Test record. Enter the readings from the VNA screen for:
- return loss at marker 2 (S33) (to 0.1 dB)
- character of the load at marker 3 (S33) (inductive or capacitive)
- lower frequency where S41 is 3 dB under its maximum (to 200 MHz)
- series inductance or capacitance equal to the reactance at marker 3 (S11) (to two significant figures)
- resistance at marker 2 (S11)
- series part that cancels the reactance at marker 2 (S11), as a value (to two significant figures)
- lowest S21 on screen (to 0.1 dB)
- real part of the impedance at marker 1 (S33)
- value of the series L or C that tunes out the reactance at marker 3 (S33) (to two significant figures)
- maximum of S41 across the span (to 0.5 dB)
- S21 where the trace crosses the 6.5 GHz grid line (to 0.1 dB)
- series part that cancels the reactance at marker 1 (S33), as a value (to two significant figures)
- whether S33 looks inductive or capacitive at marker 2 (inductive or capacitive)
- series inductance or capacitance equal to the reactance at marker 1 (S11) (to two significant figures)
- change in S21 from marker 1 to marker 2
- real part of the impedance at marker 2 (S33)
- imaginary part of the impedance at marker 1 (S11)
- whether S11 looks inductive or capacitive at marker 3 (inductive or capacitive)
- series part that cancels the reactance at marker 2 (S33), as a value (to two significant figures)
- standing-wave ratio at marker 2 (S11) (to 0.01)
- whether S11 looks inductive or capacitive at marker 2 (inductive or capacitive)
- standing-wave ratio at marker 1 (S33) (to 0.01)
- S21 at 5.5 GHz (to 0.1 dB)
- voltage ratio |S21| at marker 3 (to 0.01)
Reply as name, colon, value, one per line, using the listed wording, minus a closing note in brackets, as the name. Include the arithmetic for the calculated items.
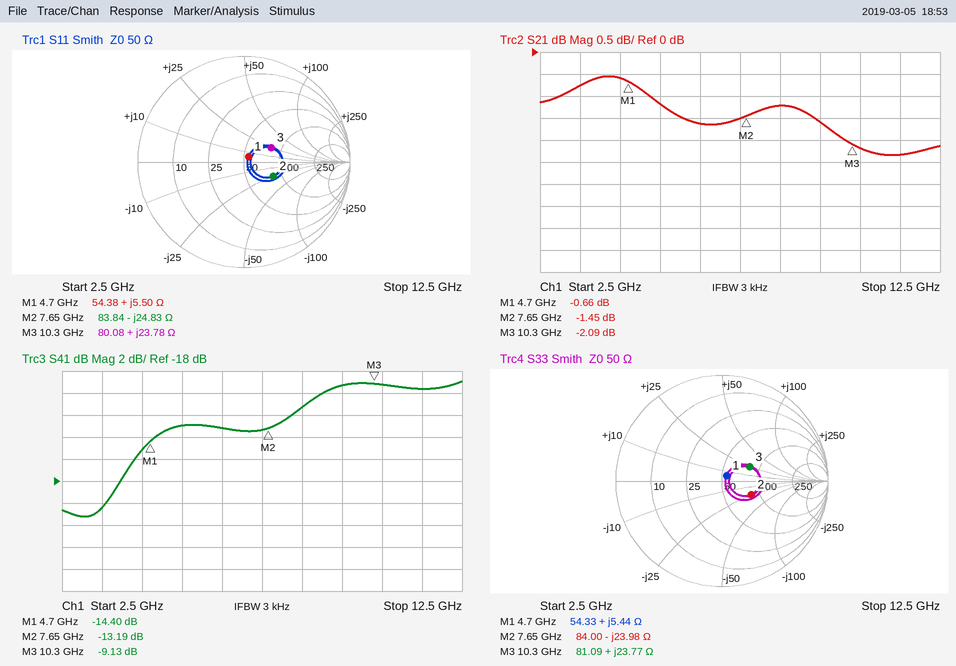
return loss at marker 2 (S33): 10.3 dB
character of the load at marker 3 (S33): inductive
lower frequency where S41 is 3 dB under its maximum: 8.2 GHz
series inductance or capacitance equal to the reactance at marker 3 (S11): L = 23.78 Ω/(2π × 10.3 GHz) ≈ 367 pH, so 370 pH to two significant figures
resistance at marker 2: 83.84 Ω
series part that cancels the reactance at marker 2 (S11), as a value: L = 24.83 Ω/(2π × 7.65 GHz) ≈ 517 pH, so 520 pH to two significant figures
lowest S21 on screen: -2.3 dB
real part of the impedance at marker 1: 54.33 Ω
value of the series L or C that tunes out the reactance at marker 3 (S33): C = 1/(2π × 10.3 GHz × 23.77 Ω) ≈ 650 fF
maximum of S41 across the span: -9.0 dB
S21 where the trace crosses the 6.5 GHz grid line: -1.6 dB
series part that cancels the reactance at marker 1 (S33), as a value: C = 1/(2π × 4.7 GHz × 5.44 Ω) ≈ 6.2 pF
whether S33 looks inductive or capacitive at marker 2: capacitive
series inductance or capacitance equal to the reactance at marker 1 (S11): L = 5.5 Ω/(2π × 4.7 GHz) ≈ 186 pH, so 190 pH to two significant figures
change in S21 from marker 1 to marker 2: -1.45 − (-0.66) = -0.79 dB
real part of the impedance at marker 2: 84.00 Ω
imaginary part of the impedance at marker 1: +5.50 Ω
whether S11 looks inductive or capacitive at marker 3: inductive
series part that cancels the reactance at marker 2 (S33), as a value: L = 23.98 Ω/(2π × 7.65 GHz) ≈ 499 pH, so 500 pH to two significant figures
standing-wave ratio at marker 2 (S11): 1.89
whether S11 looks inductive or capacitive at marker 2: capacitive
standing-wave ratio at marker 1 (S33): 1.14
S21 at 5.5 GHz: -1.2 dB
voltage ratio |S21| at marker 3: 10^(-2.09/20) ≈ 0.79
